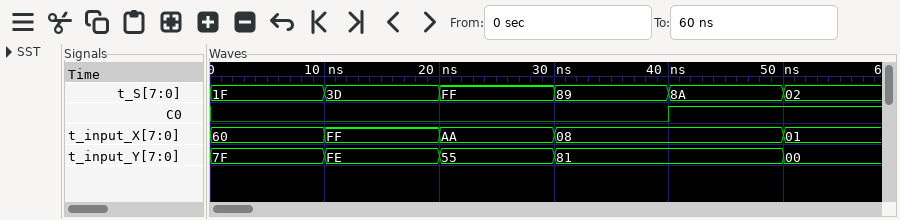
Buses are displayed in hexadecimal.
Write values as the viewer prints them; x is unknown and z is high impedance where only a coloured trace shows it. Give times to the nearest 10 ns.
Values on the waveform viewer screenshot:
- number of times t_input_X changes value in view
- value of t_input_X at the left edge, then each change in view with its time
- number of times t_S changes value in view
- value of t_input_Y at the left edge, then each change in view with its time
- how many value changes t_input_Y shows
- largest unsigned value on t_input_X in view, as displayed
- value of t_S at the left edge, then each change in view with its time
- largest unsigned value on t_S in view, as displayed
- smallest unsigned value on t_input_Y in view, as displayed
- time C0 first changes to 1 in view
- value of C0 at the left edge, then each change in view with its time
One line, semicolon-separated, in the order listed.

4; 60, FF at 10 ns, AA at 20 ns, 08 at 30 ns, 01 at 50 ns; 5; 7F, FE at 10 ns, 55 at 20 ns, 81 at 30 ns, 00 at 50 ns; 4; FF; 1F, 3D at 10 ns, FF at 20 ns, 89 at 30 ns, 8A at 40 ns, 02 at 50 ns; FF; 00; 40 ns; 0, 1 at 40 ns
